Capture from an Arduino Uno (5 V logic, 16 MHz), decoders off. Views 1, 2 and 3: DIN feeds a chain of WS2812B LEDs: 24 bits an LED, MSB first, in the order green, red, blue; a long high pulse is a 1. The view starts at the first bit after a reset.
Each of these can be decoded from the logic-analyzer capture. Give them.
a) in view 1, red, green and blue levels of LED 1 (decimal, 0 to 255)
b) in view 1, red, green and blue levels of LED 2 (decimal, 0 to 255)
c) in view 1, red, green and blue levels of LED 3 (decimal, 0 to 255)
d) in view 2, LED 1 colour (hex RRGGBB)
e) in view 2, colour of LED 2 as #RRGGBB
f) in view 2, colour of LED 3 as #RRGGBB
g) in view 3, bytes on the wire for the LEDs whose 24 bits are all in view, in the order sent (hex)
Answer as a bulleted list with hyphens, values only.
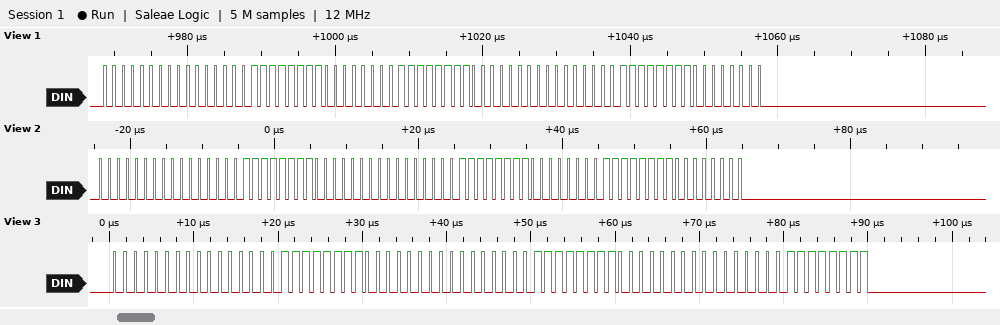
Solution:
- 0, 0, 255
- 255, 0, 0
- 255, 0, 0
- #0000FF
- #0000FF
- #FF0000
- 00 00 FF 00 00 FF 00 00 FF
